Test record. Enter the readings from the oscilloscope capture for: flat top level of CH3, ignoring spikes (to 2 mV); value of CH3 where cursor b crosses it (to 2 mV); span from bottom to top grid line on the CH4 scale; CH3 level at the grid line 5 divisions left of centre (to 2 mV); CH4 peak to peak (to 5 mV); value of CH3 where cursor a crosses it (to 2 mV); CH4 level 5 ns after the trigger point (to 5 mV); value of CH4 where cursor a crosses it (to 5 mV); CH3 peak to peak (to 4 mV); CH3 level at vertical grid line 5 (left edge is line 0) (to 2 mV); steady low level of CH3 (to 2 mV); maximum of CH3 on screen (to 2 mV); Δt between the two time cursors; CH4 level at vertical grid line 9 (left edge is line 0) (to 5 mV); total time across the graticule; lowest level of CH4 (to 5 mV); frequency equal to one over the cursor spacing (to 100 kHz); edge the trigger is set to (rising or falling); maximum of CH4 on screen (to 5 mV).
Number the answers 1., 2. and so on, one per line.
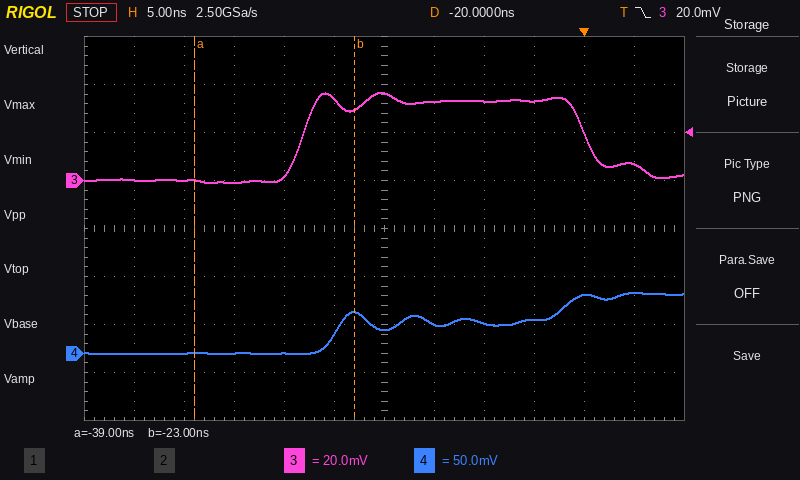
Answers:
1. 34 mV
2. 30 mV
3. 400 mV
4. 0 mV
5. 65 mV
6. 0 mV
7. 65 mV
8. 0 mV
9. 36 mV
10. 34 mV
11. 0 mV
12. 36 mV
13. 16.0 ns
14. 35 mV
15. 60 ns
16. 0 mV
17. 62.5 MHz
18. falling
19. 65 mV
